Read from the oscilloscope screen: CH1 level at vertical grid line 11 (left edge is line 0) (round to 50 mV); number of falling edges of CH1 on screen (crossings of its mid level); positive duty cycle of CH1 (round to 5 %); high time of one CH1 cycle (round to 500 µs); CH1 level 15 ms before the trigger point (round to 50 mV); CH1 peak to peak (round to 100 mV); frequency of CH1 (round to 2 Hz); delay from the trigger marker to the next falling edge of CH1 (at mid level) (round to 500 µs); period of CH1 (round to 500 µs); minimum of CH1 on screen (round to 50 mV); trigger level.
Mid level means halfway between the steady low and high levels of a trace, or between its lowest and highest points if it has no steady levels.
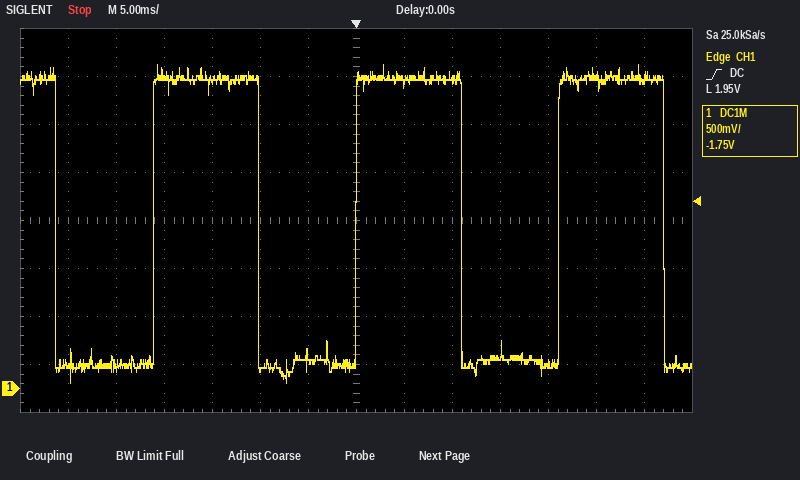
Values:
250 mV
4
50 %
11.0 ms
3.20 V
3.30 V
48 Hz
11.0 ms
21.0 ms
50 mV
1.95 V
